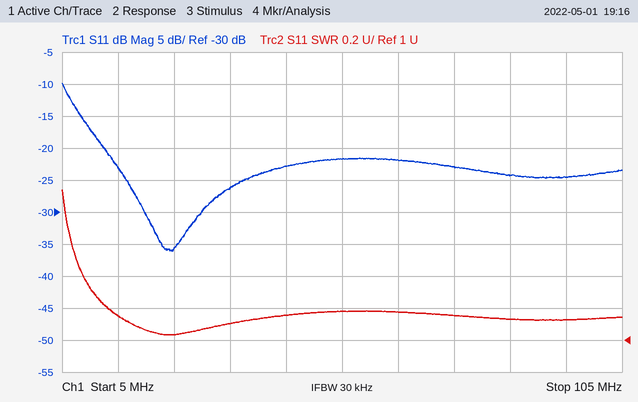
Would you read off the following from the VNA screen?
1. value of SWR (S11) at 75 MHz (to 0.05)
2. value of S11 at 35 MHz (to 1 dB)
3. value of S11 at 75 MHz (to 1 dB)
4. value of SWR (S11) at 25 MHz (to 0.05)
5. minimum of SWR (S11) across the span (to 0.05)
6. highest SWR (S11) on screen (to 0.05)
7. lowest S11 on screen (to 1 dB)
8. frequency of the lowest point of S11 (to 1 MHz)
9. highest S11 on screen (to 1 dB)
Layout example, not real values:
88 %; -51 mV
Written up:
1.15; -26 dB; -23 dB; 1.05; 1.05; 1.95; -36 dB; 25 MHz; -10 dB
